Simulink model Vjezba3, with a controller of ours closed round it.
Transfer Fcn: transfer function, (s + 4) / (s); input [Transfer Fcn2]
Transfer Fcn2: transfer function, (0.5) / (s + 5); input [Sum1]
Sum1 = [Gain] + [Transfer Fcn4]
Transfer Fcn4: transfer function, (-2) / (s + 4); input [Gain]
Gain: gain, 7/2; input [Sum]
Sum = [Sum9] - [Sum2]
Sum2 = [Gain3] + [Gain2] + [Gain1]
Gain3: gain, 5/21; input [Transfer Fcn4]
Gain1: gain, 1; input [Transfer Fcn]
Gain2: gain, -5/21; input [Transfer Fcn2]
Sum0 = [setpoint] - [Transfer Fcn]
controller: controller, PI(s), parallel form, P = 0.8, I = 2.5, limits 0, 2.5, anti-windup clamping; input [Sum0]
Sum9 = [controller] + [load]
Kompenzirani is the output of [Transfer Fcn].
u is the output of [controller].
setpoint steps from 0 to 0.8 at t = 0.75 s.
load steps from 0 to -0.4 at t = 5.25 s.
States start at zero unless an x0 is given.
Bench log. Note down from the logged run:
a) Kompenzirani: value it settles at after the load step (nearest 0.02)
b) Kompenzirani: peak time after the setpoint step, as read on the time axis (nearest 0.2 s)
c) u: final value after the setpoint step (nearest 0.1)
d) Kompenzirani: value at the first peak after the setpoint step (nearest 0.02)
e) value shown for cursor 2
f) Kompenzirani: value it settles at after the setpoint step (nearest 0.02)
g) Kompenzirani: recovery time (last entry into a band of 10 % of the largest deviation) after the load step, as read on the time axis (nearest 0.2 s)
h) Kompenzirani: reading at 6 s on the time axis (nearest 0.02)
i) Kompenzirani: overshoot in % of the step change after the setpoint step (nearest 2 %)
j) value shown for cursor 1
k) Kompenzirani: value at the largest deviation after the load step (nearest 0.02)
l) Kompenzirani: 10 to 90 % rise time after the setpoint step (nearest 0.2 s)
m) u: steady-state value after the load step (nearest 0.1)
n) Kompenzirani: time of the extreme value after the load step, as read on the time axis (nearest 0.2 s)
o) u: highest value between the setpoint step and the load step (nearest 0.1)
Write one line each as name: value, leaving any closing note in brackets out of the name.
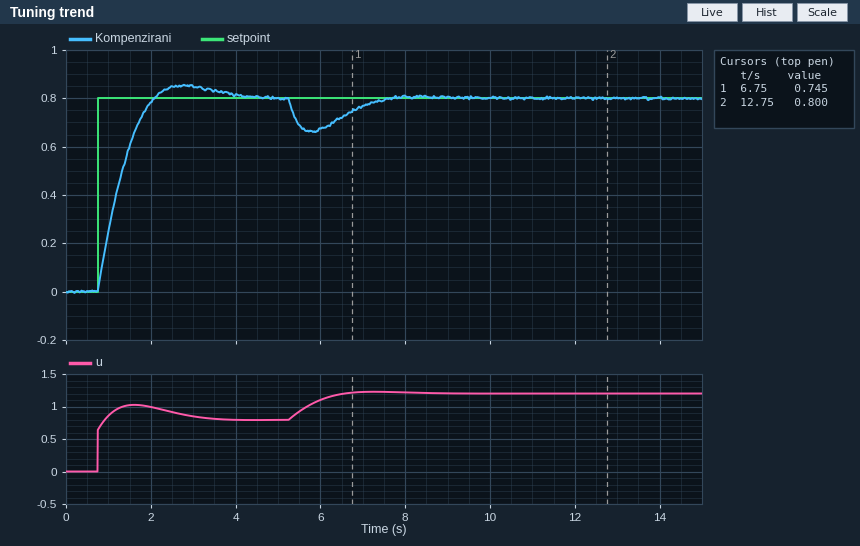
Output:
Kompenzirani: value it settles at after the load step: 0.80
Kompenzirani: peak time after the setpoint step, as read on the time axis: 2.8 s
u: final value after the setpoint step: 0.8
Kompenzirani: value at the first peak after the setpoint step: 0.86
value shown for cursor 2: 0.800
Kompenzirani: value it settles at after the setpoint step: 0.80
Kompenzirani: recovery time (last entry into a band of 10 % of the largest deviation) after the load step, as read on the time axis: 7.4 s
Kompenzirani: reading at 6 s on the time axis: 0.68
Kompenzirani: overshoot in % of the step change after the setpoint step: 6 %
value shown for cursor 1: 0.745
Kompenzirani: value at the largest deviation after the load step: 0.66
Kompenzirani: 10 to 90 % rise time after the setpoint step: 1.0 s
u: steady-state value after the load step: 1.2
Kompenzirani: time of the extreme value after the load step, as read on the time axis: 5.8 s
u: highest value between the setpoint step and the load step: 1.0
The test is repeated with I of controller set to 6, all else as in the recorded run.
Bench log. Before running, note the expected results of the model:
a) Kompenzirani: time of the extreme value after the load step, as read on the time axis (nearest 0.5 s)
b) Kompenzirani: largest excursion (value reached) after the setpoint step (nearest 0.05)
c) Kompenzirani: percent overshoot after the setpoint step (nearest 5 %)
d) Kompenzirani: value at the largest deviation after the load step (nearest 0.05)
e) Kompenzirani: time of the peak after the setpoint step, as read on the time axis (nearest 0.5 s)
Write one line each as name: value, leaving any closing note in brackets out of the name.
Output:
Kompenzirani: time of the extreme value after the load step, as read on the time axis: 5.5 s
Kompenzirani: largest excursion (value reached) after the setpoint step: 0.95
Kompenzirani: percent overshoot after the setpoint step: 20 %
Kompenzirani: value at the largest deviation after the load step: 0.70
Kompenzirani: time of the peak after the setpoint step, as read on the time axis: 2.0 s
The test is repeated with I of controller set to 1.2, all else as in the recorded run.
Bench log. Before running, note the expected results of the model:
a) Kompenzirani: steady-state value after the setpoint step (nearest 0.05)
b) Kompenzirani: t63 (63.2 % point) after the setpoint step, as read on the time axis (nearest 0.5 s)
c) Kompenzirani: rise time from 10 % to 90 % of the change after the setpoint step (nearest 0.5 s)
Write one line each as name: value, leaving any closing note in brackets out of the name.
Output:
Kompenzirani: steady-state value after the setpoint step: 0.80
Kompenzirani: t63 (63.2 % point) after the setpoint step, as read on the time axis: 1.5 s
Kompenzirani: rise time from 10 % to 90 % of the change after the setpoint step: 2.0 s
